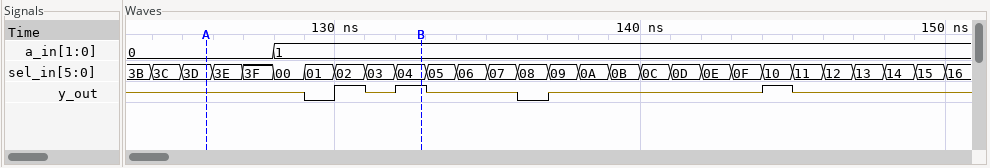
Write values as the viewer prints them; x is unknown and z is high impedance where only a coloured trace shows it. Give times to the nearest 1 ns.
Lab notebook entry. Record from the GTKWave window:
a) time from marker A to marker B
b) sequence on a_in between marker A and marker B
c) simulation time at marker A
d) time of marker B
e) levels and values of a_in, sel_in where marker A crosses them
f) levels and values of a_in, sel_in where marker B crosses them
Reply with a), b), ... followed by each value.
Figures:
a) 7 ns
b) 0, 1
c) 126 ns
d) 133 ns
e) a_in=0, sel_in=3D
f) a_in=1, sel_in=04
